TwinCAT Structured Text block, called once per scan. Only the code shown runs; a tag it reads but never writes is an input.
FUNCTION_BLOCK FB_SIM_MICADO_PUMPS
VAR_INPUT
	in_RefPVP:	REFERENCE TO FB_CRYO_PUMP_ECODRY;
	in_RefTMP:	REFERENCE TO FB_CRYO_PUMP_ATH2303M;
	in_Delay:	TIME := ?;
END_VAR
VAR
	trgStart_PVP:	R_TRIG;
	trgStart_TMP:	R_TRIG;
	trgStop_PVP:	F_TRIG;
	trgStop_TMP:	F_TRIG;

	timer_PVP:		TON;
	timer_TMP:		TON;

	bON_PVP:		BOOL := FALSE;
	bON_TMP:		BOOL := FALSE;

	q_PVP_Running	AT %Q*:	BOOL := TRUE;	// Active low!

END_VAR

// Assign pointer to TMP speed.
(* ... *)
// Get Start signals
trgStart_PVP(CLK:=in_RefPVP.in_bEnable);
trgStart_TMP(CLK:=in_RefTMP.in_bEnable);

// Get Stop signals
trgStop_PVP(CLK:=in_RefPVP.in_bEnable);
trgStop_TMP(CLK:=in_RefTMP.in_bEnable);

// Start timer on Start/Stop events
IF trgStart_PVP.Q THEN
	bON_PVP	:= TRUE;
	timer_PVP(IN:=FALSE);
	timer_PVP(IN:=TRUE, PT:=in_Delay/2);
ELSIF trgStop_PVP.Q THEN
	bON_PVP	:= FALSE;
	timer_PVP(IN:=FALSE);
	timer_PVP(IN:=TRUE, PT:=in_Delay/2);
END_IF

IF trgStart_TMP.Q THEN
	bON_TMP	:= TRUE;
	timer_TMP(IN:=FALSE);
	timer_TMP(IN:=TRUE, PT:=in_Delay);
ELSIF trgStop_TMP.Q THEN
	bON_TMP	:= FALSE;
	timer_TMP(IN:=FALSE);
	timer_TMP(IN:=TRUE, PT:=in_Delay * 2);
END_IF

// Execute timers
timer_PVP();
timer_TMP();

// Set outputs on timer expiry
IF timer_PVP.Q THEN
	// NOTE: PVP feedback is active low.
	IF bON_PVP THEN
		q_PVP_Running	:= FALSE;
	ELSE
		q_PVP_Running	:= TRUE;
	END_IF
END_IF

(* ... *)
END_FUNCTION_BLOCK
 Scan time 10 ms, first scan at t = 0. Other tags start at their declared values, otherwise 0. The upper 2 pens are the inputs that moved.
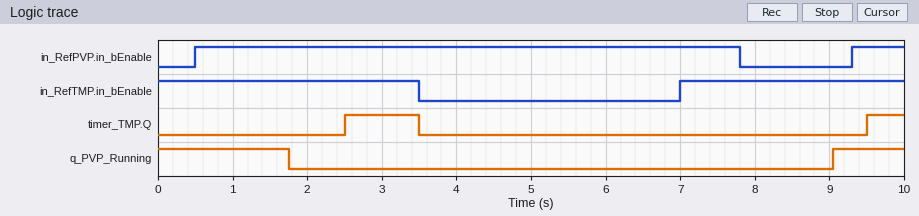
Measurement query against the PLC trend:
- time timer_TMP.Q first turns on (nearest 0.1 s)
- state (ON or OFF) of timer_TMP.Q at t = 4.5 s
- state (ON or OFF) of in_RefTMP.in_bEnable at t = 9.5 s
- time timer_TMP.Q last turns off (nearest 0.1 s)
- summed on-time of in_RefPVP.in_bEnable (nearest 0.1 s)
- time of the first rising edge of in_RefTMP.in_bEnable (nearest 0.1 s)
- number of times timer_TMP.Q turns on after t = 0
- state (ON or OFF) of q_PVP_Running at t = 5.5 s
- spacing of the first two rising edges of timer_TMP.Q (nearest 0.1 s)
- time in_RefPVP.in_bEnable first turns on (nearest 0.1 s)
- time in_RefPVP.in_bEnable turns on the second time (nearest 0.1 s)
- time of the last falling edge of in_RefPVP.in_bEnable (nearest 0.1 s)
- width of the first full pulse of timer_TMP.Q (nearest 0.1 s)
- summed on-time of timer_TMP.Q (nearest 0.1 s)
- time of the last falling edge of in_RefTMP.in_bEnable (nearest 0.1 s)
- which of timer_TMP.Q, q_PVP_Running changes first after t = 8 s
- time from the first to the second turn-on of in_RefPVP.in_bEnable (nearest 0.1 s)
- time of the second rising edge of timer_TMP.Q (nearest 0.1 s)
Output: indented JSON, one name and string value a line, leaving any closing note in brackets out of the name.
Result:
{
  "time timer_TMP.Q first turns on": "2.5 s",
  "state (ON or OFF) of timer_TMP.Q at t = 4.5 s": "OFF",
  "state (ON or OFF) of in_RefTMP.in_bEnable at t = 9.5 s": "ON",
  "time timer_TMP.Q last turns off": "3.5 s",
  "summed on-time of in_RefPVP.in_bEnable": "8.0 s",
  "time of the first rising edge of in_RefTMP.in_bEnable": "7.0 s",
  "number of times timer_TMP.Q turns on after t = 0": "2",
  "state (ON or OFF) of q_PVP_Running at t = 5.5 s": "OFF",
  "spacing of the first two rising edges of timer_TMP.Q": "7.0 s",
  "time in_RefPVP.in_bEnable first turns on": "0.5 s",
  "time in_RefPVP.in_bEnable turns on the second time": "9.3 s",
  "time of the last falling edge of in_RefPVP.in_bEnable": "7.8 s",
  "width of the first full pulse of timer_TMP.Q": "1.0 s",
  "summed on-time of timer_TMP.Q": "1.5 s",
  "time of the last falling edge of in_RefTMP.in_bEnable": "3.5 s",
  "which of timer_TMP.Q, q_PVP_Running changes first after t = 8 s": "q_PVP_Running",
  "time from the first to the second turn-on of in_RefPVP.in_bEnable": "8.8 s",
  "time of the second rising edge of timer_TMP.Q": "9.5 s"
}
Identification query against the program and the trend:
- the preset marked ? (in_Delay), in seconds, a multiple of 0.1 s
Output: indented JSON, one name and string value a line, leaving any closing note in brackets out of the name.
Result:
{
  "the preset marked ? (in_Delay), in seconds, a multiple of 0.1 s": "2.5 s"
}
